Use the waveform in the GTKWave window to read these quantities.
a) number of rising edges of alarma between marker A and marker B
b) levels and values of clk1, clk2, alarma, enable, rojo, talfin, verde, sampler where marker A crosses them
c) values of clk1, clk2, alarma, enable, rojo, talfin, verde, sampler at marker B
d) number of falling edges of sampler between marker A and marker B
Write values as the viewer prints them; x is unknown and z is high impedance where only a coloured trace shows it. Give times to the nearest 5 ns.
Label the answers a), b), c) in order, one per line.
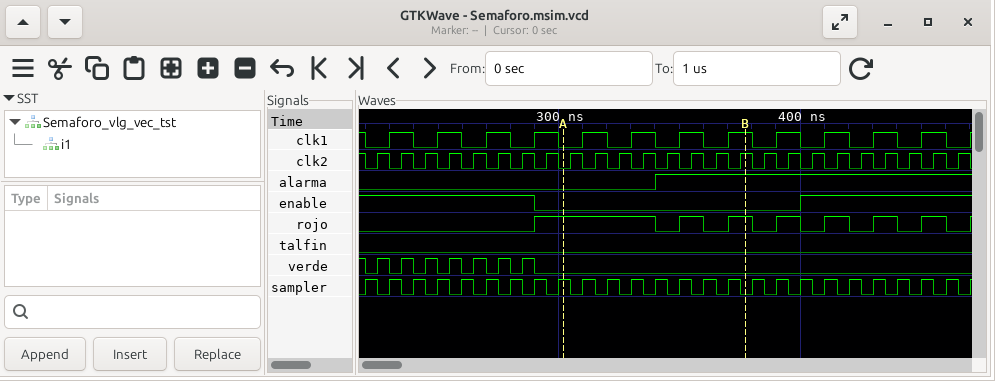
a) 1
b) clk1=0, clk2=0, alarma=0, enable=0, rojo=1, talfin=0, verde=0, sampler=1
c) clk1=1, clk2=1, alarma=1, enable=0, rojo=1, talfin=0, verde=0, sampler=0
d) 8
